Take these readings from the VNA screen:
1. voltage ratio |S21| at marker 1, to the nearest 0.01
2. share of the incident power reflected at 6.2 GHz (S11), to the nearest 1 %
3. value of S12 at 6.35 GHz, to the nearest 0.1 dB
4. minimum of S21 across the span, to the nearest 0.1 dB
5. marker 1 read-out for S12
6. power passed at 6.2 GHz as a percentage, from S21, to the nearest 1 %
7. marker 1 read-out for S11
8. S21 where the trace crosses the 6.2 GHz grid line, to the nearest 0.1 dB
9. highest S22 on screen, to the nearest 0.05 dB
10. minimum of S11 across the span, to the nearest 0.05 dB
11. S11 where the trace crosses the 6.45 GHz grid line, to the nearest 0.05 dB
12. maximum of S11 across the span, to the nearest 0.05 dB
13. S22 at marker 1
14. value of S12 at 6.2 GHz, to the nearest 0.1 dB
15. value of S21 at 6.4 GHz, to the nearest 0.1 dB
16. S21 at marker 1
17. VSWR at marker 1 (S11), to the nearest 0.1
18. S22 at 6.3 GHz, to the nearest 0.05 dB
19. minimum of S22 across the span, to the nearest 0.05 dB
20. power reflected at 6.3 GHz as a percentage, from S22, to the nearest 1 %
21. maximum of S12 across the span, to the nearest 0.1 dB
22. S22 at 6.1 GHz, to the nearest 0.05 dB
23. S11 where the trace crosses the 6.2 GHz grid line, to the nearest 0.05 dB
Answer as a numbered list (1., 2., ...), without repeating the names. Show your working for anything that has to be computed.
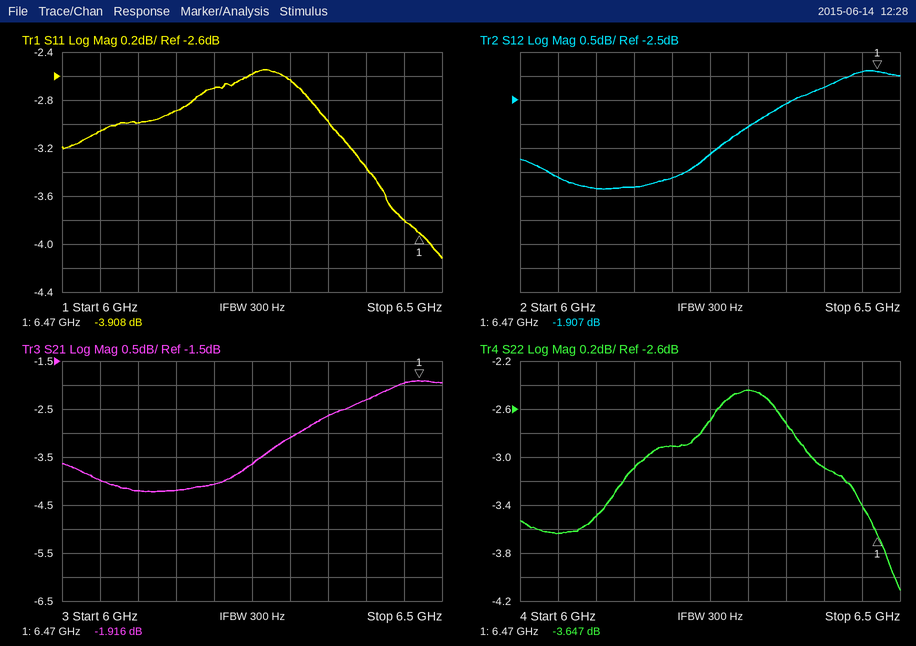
1. 10^(-1.916/20) ≈ 0.80
2. 10^(-2.7/10) ≈ 54 %
3. -2.6 dB
4. -4.2 dB
5. -1.907 dB
6. 10^(-4.1/10) ≈ 39 %
7. -3.908 dB
8. -4.1 dB
9. -2.45 dB
10. -4.10 dB
11. -3.80 dB
12. -2.55 dB
13. -3.647 dB
14. -4.1 dB
15. -2.3 dB
16. -1.916 dB
17. (1 + 0.6377)/(1 − 0.6377) ≈ 4.5
18. -2.45 dB
19. -4.10 dB
20. 10^(-2.45/10) ≈ 57 %
21. -1.9 dB
22. -3.50 dB
23. -2.70 dB
